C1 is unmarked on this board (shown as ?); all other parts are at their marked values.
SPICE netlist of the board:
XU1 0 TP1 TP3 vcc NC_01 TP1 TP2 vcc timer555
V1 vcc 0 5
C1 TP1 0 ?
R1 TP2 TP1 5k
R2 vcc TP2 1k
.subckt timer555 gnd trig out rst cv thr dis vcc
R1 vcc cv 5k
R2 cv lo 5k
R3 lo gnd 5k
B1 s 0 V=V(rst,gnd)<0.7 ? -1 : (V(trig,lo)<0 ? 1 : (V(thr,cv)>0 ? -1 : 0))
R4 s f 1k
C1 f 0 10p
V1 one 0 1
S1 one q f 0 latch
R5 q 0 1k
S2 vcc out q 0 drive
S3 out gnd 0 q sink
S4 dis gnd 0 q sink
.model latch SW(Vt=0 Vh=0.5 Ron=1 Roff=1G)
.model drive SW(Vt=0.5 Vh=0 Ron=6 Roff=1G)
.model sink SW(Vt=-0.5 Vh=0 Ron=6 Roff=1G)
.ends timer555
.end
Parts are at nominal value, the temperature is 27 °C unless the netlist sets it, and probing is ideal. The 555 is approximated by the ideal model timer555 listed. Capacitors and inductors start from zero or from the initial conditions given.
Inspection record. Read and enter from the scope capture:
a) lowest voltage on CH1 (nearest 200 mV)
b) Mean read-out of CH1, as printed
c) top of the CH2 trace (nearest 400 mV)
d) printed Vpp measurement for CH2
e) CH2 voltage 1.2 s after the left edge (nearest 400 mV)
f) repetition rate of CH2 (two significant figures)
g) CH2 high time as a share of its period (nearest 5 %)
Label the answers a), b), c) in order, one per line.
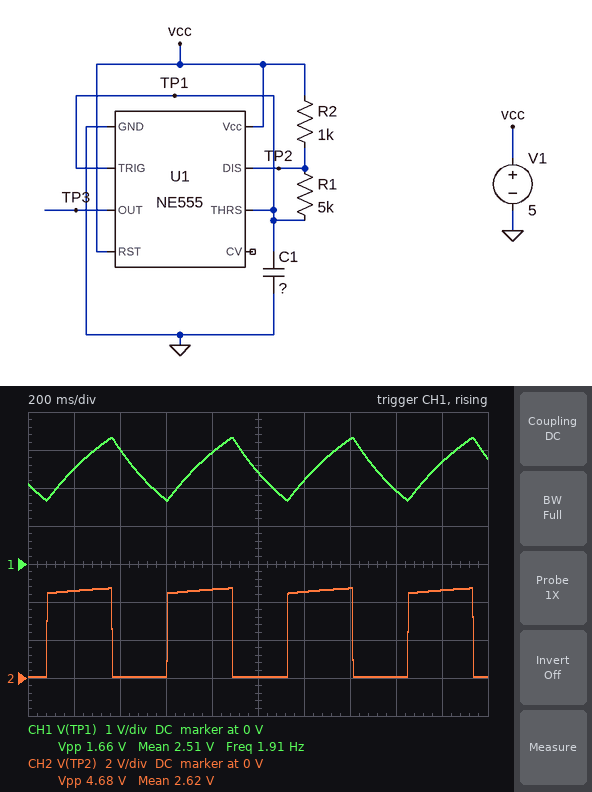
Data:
a) 1.6 V
b) 2.51 V
c) 4.8 V
d) 4.68 V
e) 4.4 V
f) 1.9 Hz
g) 55 %
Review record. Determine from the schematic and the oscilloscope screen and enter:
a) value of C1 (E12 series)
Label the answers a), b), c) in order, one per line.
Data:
a) 68 µF
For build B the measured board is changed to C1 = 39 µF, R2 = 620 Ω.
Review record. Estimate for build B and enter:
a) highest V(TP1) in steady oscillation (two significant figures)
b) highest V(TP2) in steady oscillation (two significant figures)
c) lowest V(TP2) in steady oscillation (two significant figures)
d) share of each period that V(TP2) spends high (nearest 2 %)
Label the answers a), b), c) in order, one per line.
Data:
a) 3.3 V
b) 4.8 V
c) 50 mV
d) 52 %
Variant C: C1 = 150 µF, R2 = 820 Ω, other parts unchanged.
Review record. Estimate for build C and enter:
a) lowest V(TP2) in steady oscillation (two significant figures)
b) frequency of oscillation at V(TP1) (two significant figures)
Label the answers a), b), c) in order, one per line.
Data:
a) 38 mV
b) 880 mHz
